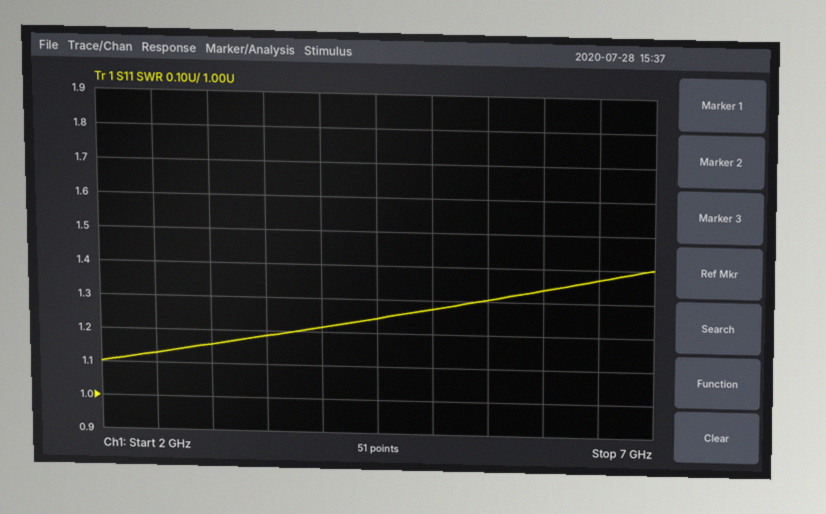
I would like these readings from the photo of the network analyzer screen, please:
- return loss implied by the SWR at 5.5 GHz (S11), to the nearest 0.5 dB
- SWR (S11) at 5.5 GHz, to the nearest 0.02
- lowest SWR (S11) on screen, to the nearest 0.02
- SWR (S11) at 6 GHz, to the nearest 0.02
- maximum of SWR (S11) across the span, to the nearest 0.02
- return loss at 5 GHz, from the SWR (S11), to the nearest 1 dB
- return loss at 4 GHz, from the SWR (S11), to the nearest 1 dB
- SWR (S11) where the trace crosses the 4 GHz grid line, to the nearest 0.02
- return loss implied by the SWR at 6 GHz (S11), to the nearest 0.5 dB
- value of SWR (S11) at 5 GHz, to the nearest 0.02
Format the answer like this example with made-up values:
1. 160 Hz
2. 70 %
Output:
1. 17.5 dB
2. 1.30
3. 1.10
4. 1.34
5. 1.40
6. 18 dB
7. 20 dB
8. 1.22
9. 17.0 dB
10. 1.28
